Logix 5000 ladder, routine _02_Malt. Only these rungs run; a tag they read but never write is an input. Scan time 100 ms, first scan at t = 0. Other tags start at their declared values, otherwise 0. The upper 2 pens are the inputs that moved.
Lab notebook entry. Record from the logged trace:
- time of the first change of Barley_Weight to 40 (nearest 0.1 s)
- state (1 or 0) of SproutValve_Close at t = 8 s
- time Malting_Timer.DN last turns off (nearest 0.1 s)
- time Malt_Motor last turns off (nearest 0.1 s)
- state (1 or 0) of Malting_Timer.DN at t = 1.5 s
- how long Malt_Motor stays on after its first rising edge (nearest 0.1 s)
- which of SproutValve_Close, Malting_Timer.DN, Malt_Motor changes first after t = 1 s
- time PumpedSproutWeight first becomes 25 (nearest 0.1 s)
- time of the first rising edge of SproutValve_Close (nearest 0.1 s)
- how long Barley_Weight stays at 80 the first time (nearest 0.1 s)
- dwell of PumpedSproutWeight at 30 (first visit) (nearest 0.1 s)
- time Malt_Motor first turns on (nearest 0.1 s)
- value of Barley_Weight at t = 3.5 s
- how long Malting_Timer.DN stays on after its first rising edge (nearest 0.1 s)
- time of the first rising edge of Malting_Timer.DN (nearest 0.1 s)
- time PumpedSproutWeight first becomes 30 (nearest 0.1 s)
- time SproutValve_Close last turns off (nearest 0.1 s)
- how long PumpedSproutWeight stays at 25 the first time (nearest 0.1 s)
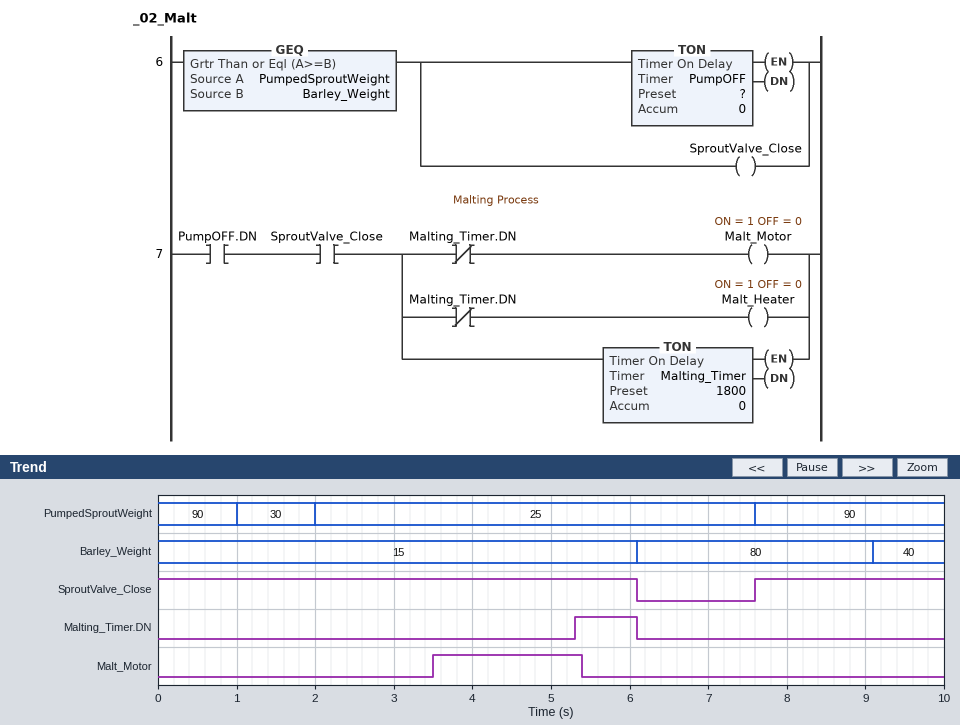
9.1 s
1
6.1 s
5.4 s
0
1.9 s
Malt_Motor
2.0 s
7.6 s
3.0 s
1.0 s
3.5 s
15
0.8 s
5.3 s
1.0 s
6.1 s
5.6 s
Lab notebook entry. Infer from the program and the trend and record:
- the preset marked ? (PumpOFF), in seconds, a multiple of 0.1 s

3.5 s
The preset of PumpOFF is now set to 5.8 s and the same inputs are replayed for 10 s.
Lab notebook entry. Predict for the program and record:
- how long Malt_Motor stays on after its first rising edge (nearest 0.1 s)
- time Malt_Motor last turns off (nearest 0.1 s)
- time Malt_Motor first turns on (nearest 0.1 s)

0.3 s
6.1 s
5.8 s
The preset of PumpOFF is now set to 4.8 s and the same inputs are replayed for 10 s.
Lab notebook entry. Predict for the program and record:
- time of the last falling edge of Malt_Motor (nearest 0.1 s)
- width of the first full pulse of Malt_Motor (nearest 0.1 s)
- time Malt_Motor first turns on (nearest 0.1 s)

6.1 s
1.3 s
4.8 s
